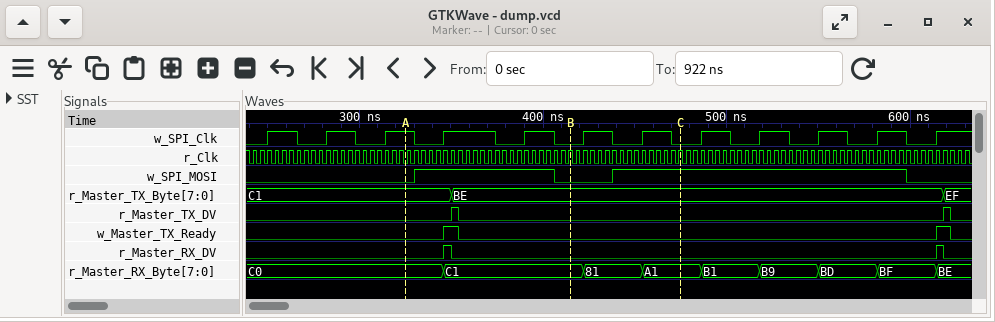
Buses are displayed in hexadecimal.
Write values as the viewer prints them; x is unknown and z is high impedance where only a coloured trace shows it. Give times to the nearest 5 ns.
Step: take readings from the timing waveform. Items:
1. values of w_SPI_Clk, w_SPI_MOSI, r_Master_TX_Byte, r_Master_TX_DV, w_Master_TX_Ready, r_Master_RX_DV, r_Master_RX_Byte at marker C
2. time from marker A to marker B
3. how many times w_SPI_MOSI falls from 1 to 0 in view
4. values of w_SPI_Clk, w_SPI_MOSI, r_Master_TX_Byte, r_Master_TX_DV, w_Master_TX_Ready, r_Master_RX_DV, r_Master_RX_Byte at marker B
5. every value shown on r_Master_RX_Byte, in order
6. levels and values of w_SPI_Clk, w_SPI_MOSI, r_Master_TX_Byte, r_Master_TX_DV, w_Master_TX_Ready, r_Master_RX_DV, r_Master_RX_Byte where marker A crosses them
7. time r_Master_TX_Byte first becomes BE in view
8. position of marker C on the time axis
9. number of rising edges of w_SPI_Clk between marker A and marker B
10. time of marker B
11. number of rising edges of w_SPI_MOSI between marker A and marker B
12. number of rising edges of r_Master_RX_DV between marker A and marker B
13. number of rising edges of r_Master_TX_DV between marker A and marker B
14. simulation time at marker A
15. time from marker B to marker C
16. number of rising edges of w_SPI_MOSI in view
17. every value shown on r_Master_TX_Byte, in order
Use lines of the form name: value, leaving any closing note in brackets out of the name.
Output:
values of w_SPI_Clk, w_SPI_MOSI, r_Master_TX_Byte, r_Master_TX_DV, w_Master_TX_Ready, r_Master_RX_DV, r_Master_RX_Byte at marker C: w_SPI_Clk=0, w_SPI_MOSI=1, r_Master_TX_Byte=BE, r_Master_TX_DV=0, w_Master_TX_Ready=0, r_Master_RX_DV=0, r_Master_RX_Byte=A1
time from marker A to marker B: 90 ns
how many times w_SPI_MOSI falls from 1 to 0 in view: 2
values of w_SPI_Clk, w_SPI_MOSI, r_Master_TX_Byte, r_Master_TX_DV, w_Master_TX_Ready, r_Master_RX_DV, r_Master_RX_Byte at marker B: w_SPI_Clk=0, w_SPI_MOSI=0, r_Master_TX_Byte=BE, r_Master_TX_DV=0, w_Master_TX_Ready=0, r_Master_RX_DV=0, r_Master_RX_Byte=C1
every value shown on r_Master_RX_Byte, in order: C0, C1, 81, A1, B1, B9, BD, BF, BE
levels and values of w_SPI_Clk, w_SPI_MOSI, r_Master_TX_Byte, r_Master_TX_DV, w_Master_TX_Ready, r_Master_RX_DV, r_Master_RX_Byte where marker A crosses them: w_SPI_Clk=1, w_SPI_MOSI=0, r_Master_TX_Byte=C1, r_Master_TX_DV=0, w_Master_TX_Ready=0, r_Master_RX_DV=0, r_Master_RX_Byte=C0
time r_Master_TX_Byte first becomes BE in view: 350 ns
position of marker C on the time axis: 475 ns
number of rising edges of w_SPI_Clk between marker A and marker B: 2
time of marker B: 415 ns
number of rising edges of w_SPI_MOSI between marker A and marker B: 1
number of rising edges of r_Master_RX_DV between marker A and marker B: 1
number of rising edges of r_Master_TX_DV between marker A and marker B: 1
simulation time at marker A: 325 ns
time from marker B to marker C: 60 ns
number of rising edges of w_SPI_MOSI in view: 2
every value shown on r_Master_TX_Byte, in order: C1, BE, EF
